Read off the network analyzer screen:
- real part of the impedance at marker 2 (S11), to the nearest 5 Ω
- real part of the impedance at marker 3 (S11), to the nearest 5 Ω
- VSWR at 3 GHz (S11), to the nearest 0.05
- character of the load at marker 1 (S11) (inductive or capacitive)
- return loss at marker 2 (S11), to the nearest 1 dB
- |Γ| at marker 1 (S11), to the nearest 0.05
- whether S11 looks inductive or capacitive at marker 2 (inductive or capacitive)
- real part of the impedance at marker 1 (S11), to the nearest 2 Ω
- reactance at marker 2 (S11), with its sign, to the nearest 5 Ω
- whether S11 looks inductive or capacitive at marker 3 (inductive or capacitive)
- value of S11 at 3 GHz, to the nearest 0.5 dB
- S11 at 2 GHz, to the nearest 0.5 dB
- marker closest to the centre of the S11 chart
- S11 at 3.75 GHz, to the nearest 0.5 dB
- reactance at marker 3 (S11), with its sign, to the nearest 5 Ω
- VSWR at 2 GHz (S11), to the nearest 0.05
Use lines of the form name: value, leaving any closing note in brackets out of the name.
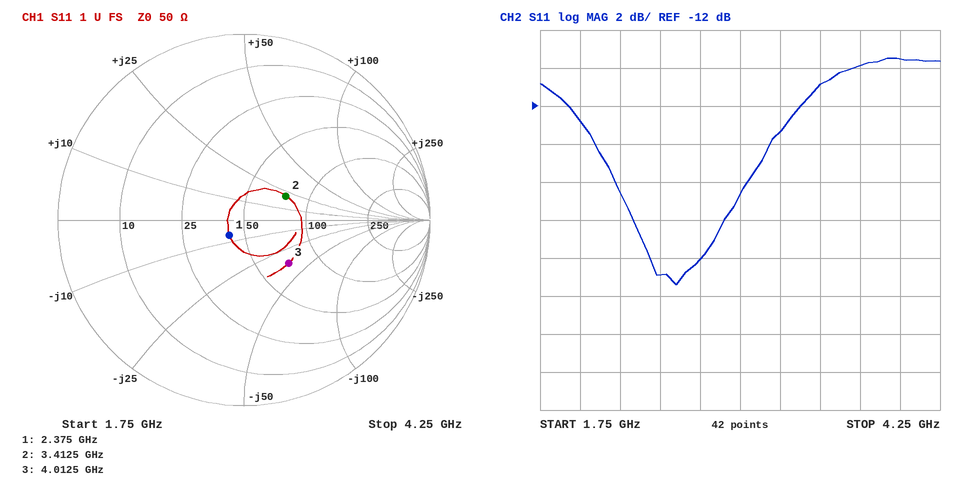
real part of the impedance at marker 2 (S11), to the nearest 5 Ω: 75 Ω
real part of the impedance at marker 3 (S11), to the nearest 5 Ω: 70 Ω
VSWR at 3 GHz (S11), to the nearest 0.05: 1.35
character of the load at marker 1 (S11): capacitive
return loss at marker 2 (S11), to the nearest 1 dB: 12 dB
|Γ| at marker 1 (S11), to the nearest 0.05: 0.10
whether S11 looks inductive or capacitive at marker 2: inductive
real part of the impedance at marker 1 (S11), to the nearest 2 Ω: 42 Ω
reactance at marker 2 (S11), with its sign, to the nearest 5 Ω: +20 Ω
whether S11 looks inductive or capacitive at marker 3: capacitive
value of S11 at 3 GHz, to the nearest 0.5 dB: -16.5 dB
S11 at 2 GHz, to the nearest 0.5 dB: -13.0 dB
marker closest to the centre of the S11 chart: marker 1
S11 at 3.75 GHz, to the nearest 0.5 dB: -10.0 dB
reactance at marker 3 (S11), with its sign, to the nearest 5 Ω: -35 Ω
VSWR at 2 GHz (S11), to the nearest 0.05: 1.60
